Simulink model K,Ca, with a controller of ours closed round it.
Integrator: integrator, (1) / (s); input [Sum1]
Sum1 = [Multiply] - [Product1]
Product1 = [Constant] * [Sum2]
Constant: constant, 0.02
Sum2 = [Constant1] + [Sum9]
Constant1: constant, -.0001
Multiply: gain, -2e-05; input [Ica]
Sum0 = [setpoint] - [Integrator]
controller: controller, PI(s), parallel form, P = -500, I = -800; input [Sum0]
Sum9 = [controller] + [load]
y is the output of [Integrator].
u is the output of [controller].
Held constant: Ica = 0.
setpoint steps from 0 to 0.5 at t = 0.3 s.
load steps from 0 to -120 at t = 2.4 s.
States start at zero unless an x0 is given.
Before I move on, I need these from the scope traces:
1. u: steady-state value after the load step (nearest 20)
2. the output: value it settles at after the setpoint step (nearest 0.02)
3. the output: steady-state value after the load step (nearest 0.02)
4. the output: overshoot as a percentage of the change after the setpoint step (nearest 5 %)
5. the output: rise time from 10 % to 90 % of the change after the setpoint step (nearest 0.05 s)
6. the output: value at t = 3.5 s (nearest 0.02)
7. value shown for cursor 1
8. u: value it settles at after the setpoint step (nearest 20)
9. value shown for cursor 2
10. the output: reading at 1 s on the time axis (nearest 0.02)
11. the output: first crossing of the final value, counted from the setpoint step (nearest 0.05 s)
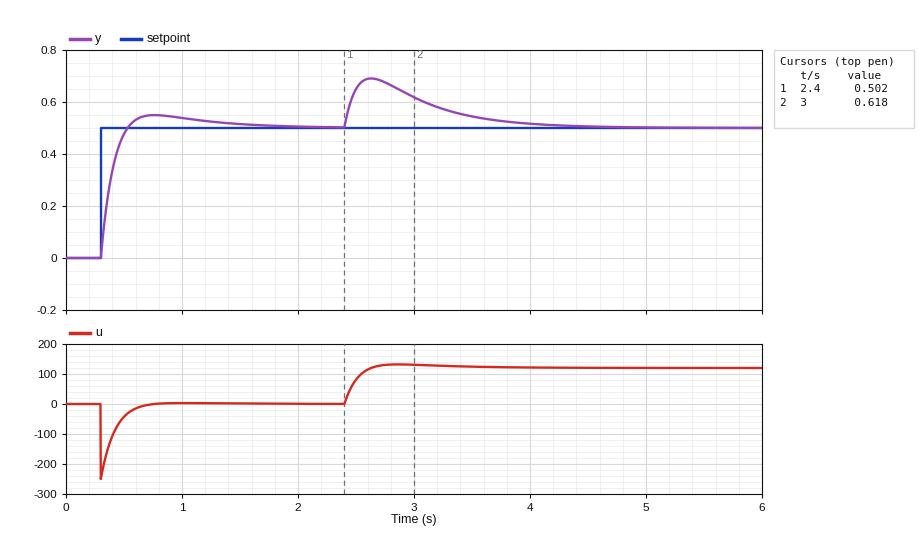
120
0.50
0.50
10 %
0.15 s
0.54
0.502
0
0.618
0.54
0.25 s
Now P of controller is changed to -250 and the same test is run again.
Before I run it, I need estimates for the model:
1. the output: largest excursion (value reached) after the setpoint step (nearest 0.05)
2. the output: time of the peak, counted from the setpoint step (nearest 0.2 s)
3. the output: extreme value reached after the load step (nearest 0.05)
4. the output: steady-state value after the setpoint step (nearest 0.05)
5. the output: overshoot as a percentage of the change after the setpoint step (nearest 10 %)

0.60
0.6 s
0.80
0.50
20 %
